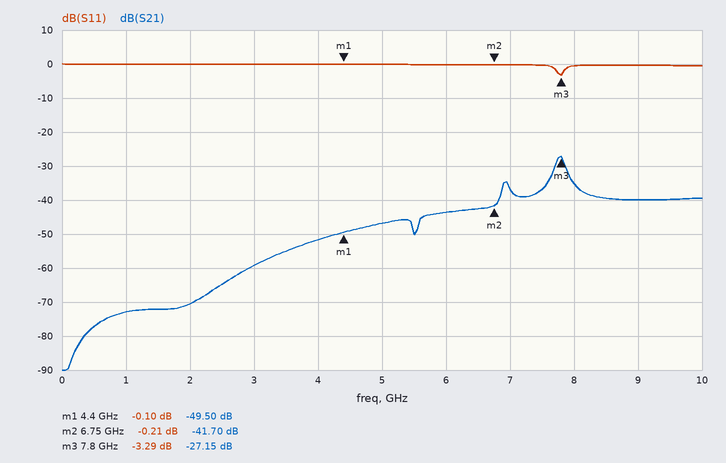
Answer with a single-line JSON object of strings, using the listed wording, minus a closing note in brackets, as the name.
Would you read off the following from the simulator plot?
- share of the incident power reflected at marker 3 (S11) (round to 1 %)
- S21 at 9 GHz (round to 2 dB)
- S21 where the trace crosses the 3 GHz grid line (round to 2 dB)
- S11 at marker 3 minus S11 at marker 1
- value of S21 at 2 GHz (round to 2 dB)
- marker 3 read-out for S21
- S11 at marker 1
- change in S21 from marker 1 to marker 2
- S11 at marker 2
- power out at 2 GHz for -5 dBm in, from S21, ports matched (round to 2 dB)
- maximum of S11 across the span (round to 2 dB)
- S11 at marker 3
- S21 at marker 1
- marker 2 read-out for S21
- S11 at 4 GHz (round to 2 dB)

{"share of the incident power reflected at marker 3 (S11)": "47 %", "S21 at 9 GHz": "-40 dB", "S21 where the trace crosses the 3 GHz grid line": "-60 dB", "S11 at marker 3 minus S11 at marker 1": "-3.19 dB", "value of S21 at 2 GHz": "-70 dB", "marker 3 read-out for S21": "-27.15 dB", "S11 at marker 1": "-0.10 dB", "change in S21 from marker 1 to marker 2": "7.80 dB", "S11 at marker 2": "-0.21 dB", "power out at 2 GHz for -5 dBm in, from S21, ports matched": "-76 dBm", "maximum of S11 across the span": "0 dB", "S11 at marker 3": "-3.29 dB", "S21 at marker 1": "-49.50 dB", "marker 2 read-out for S21": "-41.70 dB", "S11 at 4 GHz": "0 dB"}
